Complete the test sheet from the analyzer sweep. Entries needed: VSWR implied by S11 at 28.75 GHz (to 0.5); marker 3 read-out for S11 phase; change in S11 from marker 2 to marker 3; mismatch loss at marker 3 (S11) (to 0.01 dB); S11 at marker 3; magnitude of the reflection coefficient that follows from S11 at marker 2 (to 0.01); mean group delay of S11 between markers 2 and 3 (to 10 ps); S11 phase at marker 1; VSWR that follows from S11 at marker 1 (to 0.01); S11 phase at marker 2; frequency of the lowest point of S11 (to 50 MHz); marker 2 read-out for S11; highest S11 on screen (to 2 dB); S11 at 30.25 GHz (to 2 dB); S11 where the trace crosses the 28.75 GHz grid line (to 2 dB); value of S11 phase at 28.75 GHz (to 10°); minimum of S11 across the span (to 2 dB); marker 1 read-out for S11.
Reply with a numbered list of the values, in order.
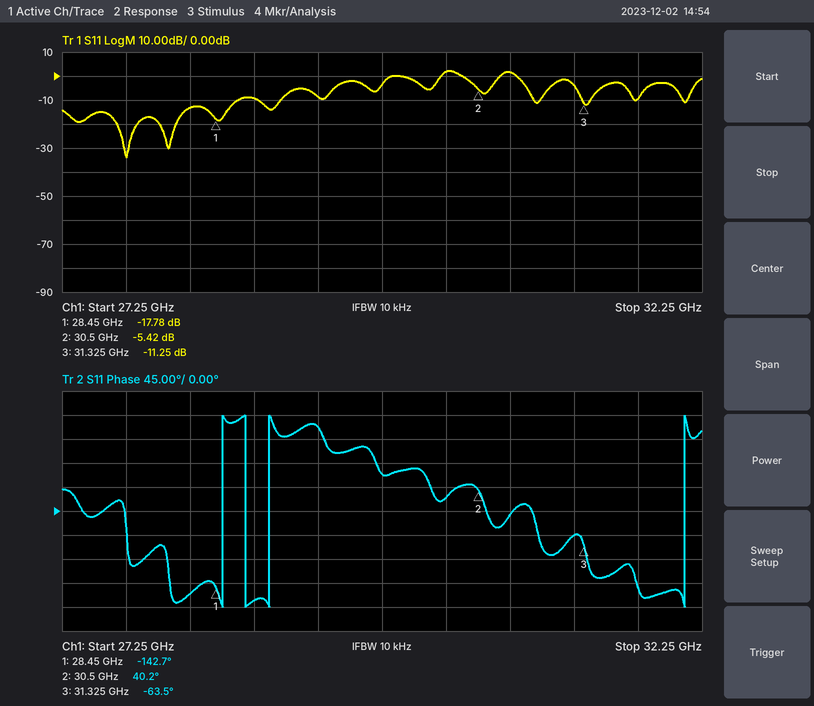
1. 2.0
2. -63.5°
3. -5.83 dB
4. 0.34 dB
5. -11.25 dB
6. 0.54
7. 350 ps
8. -142.7°
9. 1.30
10. 40.2°
11. 27.75 GHz
12. -5.42 dB
13. 2 dB
14. 2 dB
15. -10 dB
16. -170°
17. -34 dB
18. -17.78 dB
